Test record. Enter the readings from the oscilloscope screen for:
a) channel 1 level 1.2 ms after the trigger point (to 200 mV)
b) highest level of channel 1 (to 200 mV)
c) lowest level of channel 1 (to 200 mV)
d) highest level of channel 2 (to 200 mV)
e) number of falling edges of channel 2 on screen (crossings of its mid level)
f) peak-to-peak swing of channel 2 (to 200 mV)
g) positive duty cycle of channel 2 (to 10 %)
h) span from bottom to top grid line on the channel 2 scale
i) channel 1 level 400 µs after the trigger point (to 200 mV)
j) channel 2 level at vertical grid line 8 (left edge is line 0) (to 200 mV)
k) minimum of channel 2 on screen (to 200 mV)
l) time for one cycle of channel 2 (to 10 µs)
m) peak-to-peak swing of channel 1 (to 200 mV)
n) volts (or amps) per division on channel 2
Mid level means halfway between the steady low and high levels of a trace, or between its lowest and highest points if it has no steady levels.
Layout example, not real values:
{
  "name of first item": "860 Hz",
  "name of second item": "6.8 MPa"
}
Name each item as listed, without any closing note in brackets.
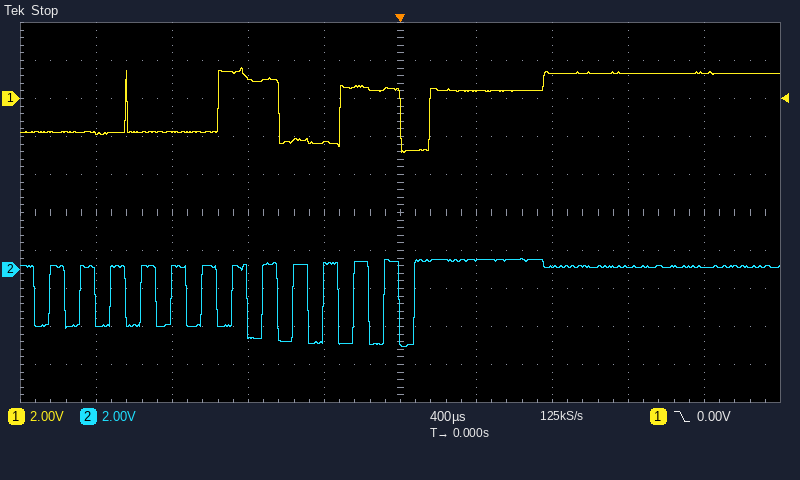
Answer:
{
  "channel 1 level 1.2 ms after the trigger point": "1.4 V",
  "highest level of channel 1": "1.6 V",
  "lowest level of channel 1": "-2.8 V",
  "highest level of channel 2": "600 mV",
  "number of falling edges of channel 2 on screen": "13",
  "peak-to-peak swing of channel 2": "4.6 V",
  "positive duty cycle of channel 2": "50 %",
  "span from bottom to top grid line on the channel 2 scale": "20 V",
  "channel 1 level 400 µs after the trigger point": "400 mV",
  "channel 2 level at vertical grid line 8 (left edge is line 0)": "200 mV",
  "minimum of channel 2 on screen": "-4.0 V",
  "time for one cycle of channel 2": "160 µs",
  "peak-to-peak swing of channel 1": "4.4 V",
  "volts (or amps) per division on channel 2": "2 V"
}
